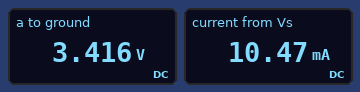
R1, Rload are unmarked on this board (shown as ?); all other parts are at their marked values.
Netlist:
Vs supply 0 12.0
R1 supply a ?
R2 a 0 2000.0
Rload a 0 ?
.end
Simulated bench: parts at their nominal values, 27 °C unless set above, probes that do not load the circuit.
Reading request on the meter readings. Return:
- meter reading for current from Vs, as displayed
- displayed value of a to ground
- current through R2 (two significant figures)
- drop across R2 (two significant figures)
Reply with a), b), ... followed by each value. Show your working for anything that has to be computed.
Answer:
a) 10.47 mA
b) 3.416 V
c) (3.416 V) / 2 kΩ = 1.7 mA
d) 3.416 V = 3.4 V
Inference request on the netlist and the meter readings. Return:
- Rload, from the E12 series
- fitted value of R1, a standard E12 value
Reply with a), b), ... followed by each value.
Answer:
a) 390 Ω
b) 820 Ω
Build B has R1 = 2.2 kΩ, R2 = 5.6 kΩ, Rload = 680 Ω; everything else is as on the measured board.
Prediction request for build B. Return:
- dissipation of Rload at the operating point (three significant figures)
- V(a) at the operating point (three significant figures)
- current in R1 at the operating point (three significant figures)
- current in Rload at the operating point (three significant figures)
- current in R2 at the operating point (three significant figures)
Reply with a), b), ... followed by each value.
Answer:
a) 9.89 mW
b) 2.59 V
c) 4.28 mA
d) 3.81 mA
e) 463 µA
